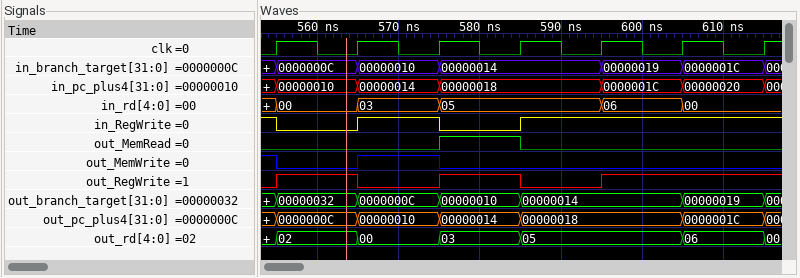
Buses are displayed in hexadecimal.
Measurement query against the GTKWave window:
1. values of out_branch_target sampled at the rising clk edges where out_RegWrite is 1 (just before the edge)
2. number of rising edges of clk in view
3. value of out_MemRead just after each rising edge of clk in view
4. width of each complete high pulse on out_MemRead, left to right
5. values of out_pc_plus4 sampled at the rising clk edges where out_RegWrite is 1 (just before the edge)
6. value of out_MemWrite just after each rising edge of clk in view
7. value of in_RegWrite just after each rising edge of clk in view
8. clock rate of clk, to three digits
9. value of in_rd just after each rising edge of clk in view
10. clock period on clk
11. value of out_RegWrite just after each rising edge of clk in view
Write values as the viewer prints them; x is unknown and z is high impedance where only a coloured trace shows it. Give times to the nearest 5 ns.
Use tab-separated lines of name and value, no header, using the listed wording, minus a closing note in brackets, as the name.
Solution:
values of out_branch_target sampled at the rising clk edges where out_RegWrite is 1	00000032, 00000010, 00000014, 00000019
number of rising edges of clk in view	7
value of out_MemRead just after each rising edge of clk in view	0 0 1 0 0 0 0
width of each complete high pulse on out_MemRead, left to right	10 ns
values of out_pc_plus4 sampled at the rising clk edges where out_RegWrite is 1	0000000C, 00000014, 00000018, 0000001C
value of out_MemWrite just after each rising edge of clk in view	0 1 0 0 0 0 0
value of in_RegWrite just after each rising edge of clk in view	0 1 0 1 1 1 1
clock rate of clk, to three digits	100 MHz
value of in_rd just after each rising edge of clk in view	00, 03, 05, 05, 06, 00, 00
clock period on clk	10 ns
value of out_RegWrite just after each rising edge of clk in view	1 0 1 0 1 1 1
